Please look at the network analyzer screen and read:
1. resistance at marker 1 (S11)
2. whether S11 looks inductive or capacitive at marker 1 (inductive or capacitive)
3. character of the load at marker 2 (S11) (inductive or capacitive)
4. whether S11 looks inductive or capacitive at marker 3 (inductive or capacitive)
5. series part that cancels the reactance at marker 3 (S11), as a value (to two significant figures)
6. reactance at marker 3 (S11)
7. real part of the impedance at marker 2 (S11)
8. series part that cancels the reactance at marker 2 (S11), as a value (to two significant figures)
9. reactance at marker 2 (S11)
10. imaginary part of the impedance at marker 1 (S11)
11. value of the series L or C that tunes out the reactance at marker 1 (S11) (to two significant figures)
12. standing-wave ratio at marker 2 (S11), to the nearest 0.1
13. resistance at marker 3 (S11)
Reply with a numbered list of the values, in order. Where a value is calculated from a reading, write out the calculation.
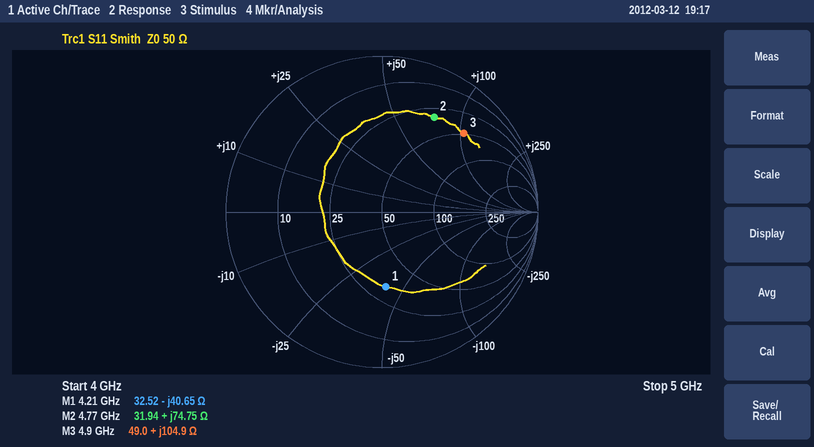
1. 32.52 Ω
2. capacitive
3. inductive
4. inductive
5. C = 1/(2π × 4.9 GHz × 104.9 Ω) ≈ 310 fF
6. +104.9 Ω
7. 31.94 Ω
8. C = 1/(2π × 4.77 GHz × 74.75 Ω) ≈ 446 fF, so 450 fF to two significant figures
9. +74.75 Ω
10. -40.65 Ω
11. L = 40.65 Ω/(2π × 4.21 GHz) ≈ 1.5 nH
12. 5.5
13. 49.0 Ω
